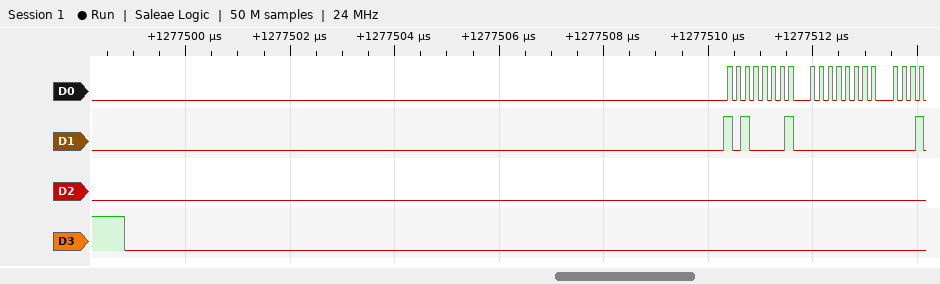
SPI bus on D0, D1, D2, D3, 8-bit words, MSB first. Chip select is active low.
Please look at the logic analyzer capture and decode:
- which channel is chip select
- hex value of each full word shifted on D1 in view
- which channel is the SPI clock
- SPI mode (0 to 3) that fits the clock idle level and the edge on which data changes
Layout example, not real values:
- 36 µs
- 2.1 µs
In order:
- D3
- A1, 00
- D0
- 0
